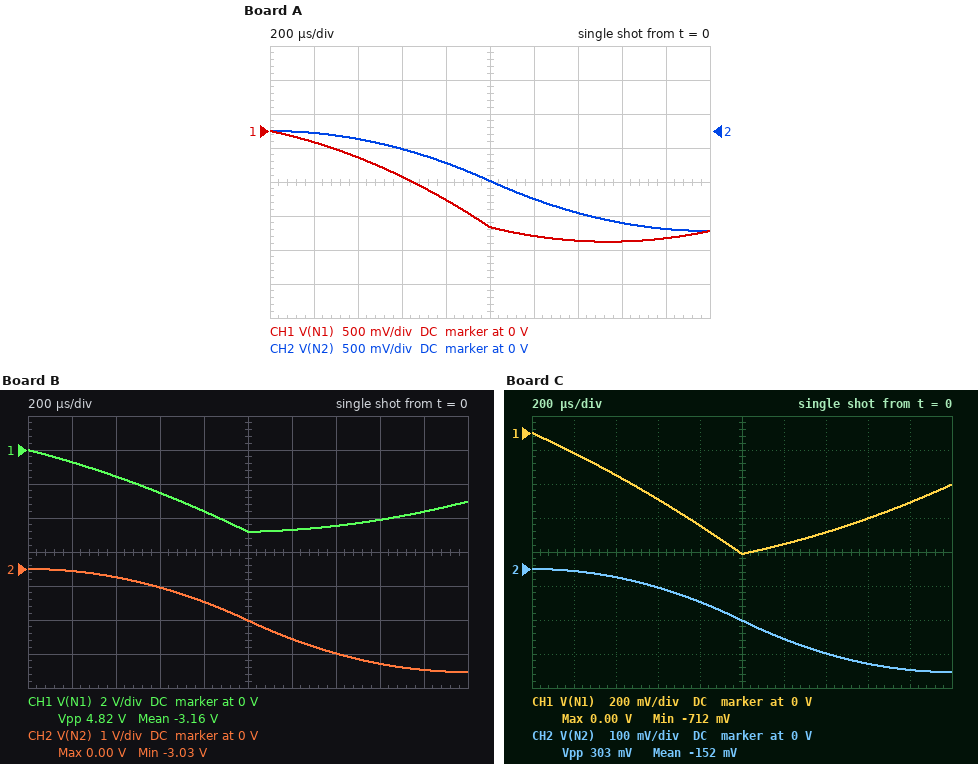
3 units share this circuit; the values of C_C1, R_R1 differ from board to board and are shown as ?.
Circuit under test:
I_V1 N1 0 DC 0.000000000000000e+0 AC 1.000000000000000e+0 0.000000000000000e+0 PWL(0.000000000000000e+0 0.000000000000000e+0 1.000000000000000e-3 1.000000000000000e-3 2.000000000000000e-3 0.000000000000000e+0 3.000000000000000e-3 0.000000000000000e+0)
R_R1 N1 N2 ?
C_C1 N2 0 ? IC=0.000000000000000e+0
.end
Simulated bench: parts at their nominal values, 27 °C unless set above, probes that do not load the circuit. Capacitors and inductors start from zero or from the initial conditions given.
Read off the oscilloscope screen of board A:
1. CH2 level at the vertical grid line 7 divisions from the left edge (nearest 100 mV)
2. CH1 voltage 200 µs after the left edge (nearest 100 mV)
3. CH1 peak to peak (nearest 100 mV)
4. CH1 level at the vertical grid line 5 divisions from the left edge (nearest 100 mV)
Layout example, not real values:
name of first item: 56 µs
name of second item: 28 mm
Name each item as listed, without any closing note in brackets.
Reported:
CH2 level at the vertical grid line 7 divisions from the left edge: -1.2 V
CH1 voltage 200 µs after the left edge: -200 mV
CH1 peak to peak: 1.6 V
CH1 level at the vertical grid line 5 divisions from the left edge: -1.4 V
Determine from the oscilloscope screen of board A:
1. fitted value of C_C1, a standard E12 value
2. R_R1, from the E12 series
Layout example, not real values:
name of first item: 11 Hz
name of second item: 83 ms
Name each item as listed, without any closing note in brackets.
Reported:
fitted value of C_C1, a standard E12 value: 680 nF
R_R1, from the E12 series: 680 Ω
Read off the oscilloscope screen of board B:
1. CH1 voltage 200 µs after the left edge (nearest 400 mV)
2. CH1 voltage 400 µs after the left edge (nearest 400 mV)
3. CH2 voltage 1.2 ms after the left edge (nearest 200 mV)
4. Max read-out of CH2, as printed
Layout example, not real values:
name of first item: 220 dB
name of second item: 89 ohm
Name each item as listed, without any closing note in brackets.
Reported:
CH1 voltage 200 µs after the left edge: -800 mV
CH1 voltage 400 µs after the left edge: -1.6 V
CH2 voltage 1.2 ms after the left edge: -2.0 V
Max read-out of CH2, as printed: 0.00 V
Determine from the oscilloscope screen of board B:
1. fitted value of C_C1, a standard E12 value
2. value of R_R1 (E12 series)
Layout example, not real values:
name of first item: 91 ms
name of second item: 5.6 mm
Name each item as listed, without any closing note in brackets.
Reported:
fitted value of C_C1, a standard E12 value: 330 nF
value of R_R1: 3.3 kΩ
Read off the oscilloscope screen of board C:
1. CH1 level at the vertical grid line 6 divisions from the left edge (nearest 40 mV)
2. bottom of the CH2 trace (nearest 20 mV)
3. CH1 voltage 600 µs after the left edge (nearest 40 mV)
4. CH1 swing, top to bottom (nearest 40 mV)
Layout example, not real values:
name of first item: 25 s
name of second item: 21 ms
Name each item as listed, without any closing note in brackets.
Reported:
CH1 level at the vertical grid line 6 divisions from the left edge: -640 mV
bottom of the CH2 trace: -300 mV
CH1 voltage 600 µs after the left edge: -400 mV
CH1 swing, top to bottom: 720 mV
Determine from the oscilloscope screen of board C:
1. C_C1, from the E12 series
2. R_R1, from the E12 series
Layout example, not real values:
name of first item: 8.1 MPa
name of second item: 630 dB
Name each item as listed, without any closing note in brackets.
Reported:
C_C1, from the E12 series: 3.3 µF
R_R1, from the E12 series: 560 Ω
